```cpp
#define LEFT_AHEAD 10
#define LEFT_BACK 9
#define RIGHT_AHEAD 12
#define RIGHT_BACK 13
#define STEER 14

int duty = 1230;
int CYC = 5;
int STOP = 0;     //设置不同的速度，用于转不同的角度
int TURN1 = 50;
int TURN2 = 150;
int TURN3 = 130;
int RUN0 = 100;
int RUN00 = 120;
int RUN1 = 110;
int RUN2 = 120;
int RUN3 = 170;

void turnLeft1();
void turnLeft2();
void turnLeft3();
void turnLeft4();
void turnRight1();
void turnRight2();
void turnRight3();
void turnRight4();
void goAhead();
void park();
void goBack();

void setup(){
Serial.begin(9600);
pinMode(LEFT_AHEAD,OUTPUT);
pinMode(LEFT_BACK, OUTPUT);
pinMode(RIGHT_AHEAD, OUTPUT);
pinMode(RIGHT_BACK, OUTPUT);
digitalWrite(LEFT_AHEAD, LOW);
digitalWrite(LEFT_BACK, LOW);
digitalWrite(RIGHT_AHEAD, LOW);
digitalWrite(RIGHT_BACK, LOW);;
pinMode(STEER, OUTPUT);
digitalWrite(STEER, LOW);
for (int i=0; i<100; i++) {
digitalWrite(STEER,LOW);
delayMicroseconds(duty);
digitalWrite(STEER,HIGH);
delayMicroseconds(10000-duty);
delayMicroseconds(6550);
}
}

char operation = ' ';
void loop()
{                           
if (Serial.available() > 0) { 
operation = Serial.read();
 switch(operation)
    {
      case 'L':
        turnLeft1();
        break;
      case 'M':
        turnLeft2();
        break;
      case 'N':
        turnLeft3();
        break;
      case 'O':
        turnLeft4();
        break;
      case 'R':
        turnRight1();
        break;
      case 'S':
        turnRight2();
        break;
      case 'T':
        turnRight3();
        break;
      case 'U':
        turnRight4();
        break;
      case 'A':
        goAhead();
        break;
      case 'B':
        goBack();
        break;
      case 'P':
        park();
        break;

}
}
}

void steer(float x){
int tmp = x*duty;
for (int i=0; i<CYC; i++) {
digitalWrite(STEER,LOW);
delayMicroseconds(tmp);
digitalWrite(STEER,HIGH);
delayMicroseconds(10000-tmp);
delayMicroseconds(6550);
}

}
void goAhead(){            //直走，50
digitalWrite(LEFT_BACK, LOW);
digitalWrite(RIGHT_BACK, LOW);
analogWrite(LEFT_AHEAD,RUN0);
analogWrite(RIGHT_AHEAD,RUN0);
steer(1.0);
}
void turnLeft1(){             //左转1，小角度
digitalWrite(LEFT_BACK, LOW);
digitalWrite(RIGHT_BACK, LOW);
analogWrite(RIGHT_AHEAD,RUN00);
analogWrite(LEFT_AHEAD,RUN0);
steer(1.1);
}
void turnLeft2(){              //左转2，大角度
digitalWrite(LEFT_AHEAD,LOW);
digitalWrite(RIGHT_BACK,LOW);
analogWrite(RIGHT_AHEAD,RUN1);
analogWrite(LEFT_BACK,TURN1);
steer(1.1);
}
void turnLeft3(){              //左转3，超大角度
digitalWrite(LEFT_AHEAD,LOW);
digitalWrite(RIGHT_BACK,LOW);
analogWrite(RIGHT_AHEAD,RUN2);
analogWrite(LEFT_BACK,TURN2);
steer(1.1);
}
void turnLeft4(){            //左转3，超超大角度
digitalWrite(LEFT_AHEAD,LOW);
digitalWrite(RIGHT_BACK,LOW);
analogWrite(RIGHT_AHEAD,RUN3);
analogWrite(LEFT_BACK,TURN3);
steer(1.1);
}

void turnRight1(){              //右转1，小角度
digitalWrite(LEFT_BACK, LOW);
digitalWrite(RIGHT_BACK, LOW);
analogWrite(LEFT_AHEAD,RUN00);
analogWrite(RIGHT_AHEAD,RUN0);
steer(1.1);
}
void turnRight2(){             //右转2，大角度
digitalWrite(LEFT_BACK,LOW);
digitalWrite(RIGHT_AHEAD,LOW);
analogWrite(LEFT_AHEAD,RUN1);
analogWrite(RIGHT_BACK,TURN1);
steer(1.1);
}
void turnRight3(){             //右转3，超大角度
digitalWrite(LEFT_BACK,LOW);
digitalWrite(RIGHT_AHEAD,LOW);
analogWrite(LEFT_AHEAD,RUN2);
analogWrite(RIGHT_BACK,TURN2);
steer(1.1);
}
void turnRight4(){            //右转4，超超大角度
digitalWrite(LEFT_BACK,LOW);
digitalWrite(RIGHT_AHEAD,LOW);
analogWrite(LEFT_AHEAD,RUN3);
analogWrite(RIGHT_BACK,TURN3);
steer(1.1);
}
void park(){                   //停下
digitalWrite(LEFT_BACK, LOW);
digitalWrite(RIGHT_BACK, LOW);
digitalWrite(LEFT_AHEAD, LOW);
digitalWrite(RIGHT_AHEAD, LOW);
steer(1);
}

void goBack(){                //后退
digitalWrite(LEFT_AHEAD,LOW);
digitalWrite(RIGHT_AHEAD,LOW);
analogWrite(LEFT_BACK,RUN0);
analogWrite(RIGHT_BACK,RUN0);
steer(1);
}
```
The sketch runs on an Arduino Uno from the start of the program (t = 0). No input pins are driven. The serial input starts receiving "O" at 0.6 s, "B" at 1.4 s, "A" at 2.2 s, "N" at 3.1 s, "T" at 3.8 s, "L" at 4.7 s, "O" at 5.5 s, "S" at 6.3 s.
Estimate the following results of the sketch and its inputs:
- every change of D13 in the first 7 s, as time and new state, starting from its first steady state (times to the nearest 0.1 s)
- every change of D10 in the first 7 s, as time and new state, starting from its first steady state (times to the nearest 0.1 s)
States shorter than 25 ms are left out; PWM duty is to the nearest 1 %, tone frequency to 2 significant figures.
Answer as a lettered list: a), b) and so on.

a) 0 s low; 3.8 s high; 4.7 s low
b) 0 s low; 2.2 s PWM 39 %; 3.1 s low; 3.8 s PWM 47 %; 4.7 s PWM 39 %; 5.5 s low; 6.3 s PWM 43 %
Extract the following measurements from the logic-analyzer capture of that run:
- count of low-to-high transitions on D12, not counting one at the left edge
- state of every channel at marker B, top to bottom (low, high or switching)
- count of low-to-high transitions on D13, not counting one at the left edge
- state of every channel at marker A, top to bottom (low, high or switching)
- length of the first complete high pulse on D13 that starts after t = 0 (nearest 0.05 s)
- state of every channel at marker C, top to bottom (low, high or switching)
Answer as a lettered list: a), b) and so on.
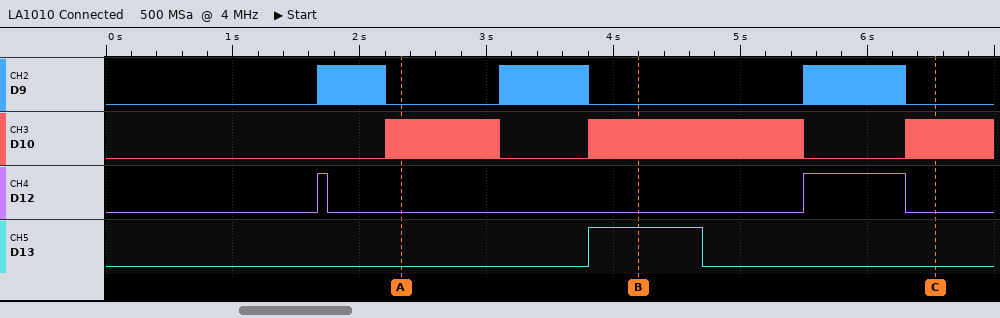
a) 2
b) D9 low, D10 switching, D12 low, D13 high
c) 1
d) D9 low, D10 switching, D12 low, D13 low
e) 0.90 s
f) D9 low, D10 switching, D12 low, D13 low
